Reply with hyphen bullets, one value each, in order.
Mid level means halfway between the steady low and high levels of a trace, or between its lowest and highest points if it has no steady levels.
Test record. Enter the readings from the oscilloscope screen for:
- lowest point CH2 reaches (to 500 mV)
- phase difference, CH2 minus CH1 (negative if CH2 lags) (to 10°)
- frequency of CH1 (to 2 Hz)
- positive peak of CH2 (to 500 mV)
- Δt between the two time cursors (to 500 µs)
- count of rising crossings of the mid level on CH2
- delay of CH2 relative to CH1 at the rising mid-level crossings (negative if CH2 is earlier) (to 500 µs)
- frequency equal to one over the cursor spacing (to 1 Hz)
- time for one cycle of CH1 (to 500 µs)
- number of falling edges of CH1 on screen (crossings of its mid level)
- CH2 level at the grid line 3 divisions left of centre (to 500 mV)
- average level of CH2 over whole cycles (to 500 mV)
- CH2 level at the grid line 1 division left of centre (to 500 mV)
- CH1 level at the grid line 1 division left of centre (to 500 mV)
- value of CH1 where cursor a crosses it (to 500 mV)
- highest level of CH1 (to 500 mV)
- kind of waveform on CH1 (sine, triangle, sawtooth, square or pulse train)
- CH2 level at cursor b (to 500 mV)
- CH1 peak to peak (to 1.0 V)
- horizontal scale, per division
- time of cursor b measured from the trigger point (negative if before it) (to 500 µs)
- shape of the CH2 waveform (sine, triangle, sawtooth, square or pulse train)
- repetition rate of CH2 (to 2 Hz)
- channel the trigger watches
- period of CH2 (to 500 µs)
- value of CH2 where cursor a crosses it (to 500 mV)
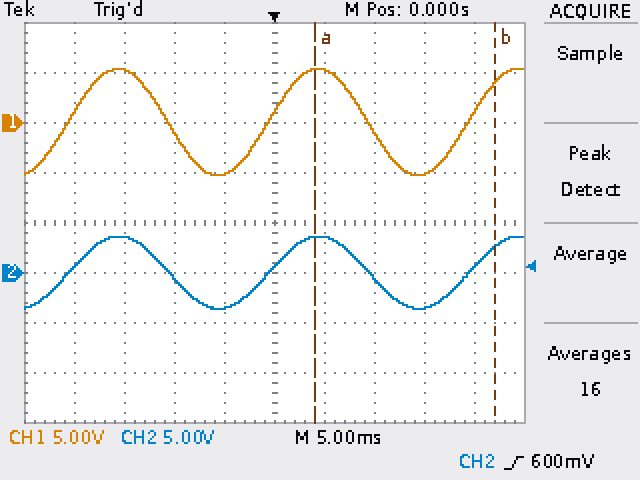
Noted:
- -3.5 V
- 0°
- 50 Hz
- 3.5 V
- 18.0 ms
- 3
- 0.0 ms
- 56 Hz
- 20.0 ms
- 2
- 3.5 V
- 0.0 V
- -3.5 V
- -5.0 V
- 5.5 V
- 5.5 V
- sine
- 2.5 V
- 11.0 V
- 5 ms
- +22.0 ms
- sine
- 50 Hz
- CH2
- 20.0 ms
- 3.5 V
